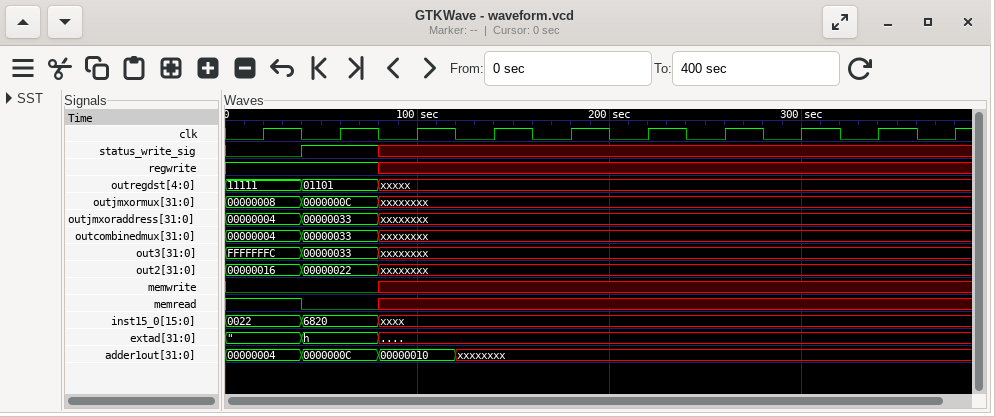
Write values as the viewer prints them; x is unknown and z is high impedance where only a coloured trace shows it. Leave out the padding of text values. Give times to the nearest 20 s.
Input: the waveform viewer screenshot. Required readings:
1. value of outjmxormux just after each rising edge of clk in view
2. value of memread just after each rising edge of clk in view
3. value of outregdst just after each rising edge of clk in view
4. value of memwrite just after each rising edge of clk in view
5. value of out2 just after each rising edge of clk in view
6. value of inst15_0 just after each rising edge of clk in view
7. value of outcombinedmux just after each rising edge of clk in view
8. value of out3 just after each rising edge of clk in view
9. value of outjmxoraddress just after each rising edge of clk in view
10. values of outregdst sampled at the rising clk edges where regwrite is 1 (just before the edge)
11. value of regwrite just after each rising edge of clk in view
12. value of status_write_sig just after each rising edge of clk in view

00000008, 0000000C, xxxxxxxx, xxxxxxxx, xxxxxxxx, xxxxxxxx, xxxxxxxx, xxxxxxxx, xxxxxxxx, xxxxxxxx
1 0 x x x x x x x x
11111, 01101, xxxxx, xxxxx, xxxxx, xxxxx, xxxxx, xxxxx, xxxxx, xxxxx
0 0 x x x x x x x x
00000016, 00000022, xxxxxxxx, xxxxxxxx, xxxxxxxx, xxxxxxxx, xxxxxxxx, xxxxxxxx, xxxxxxxx, xxxxxxxx
0022, 6820, xxxx, xxxx, xxxx, xxxx, xxxx, xxxx, xxxx, xxxx
00000004, 00000033, xxxxxxxx, xxxxxxxx, xxxxxxxx, xxxxxxxx, xxxxxxxx, xxxxxxxx, xxxxxxxx, xxxxxxxx
FFFFFFFC, 00000033, xxxxxxxx, xxxxxxxx, xxxxxxxx, xxxxxxxx, xxxxxxxx, xxxxxxxx, xxxxxxxx, xxxxxxxx
00000004, 00000033, xxxxxxxx, xxxxxxxx, xxxxxxxx, xxxxxxxx, xxxxxxxx, xxxxxxxx, xxxxxxxx, xxxxxxxx
11111, 01101
1 1 x x x x x x x x
0 1 x x x x x x x x
